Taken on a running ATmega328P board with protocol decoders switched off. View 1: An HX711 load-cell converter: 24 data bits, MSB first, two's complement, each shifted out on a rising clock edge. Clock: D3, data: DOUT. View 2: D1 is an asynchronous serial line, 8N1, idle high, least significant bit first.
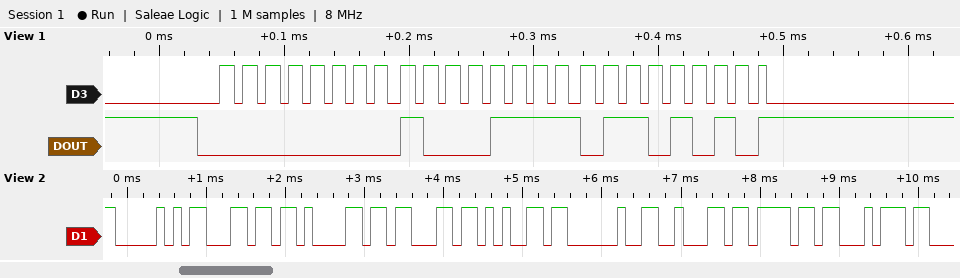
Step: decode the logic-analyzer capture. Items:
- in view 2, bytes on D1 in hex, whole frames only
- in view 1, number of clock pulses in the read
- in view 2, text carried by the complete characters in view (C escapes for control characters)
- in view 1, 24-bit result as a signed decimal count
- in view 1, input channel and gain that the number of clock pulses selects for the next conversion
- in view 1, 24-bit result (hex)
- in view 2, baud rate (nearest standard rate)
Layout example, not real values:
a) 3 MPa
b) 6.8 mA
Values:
a) 50 6C 61 63 65 20 62 6F 74
b) 25
c) "Place bot"
d) 36714
e) channel A, gain 128
f) 0x008F6A
g) 9600 baud
